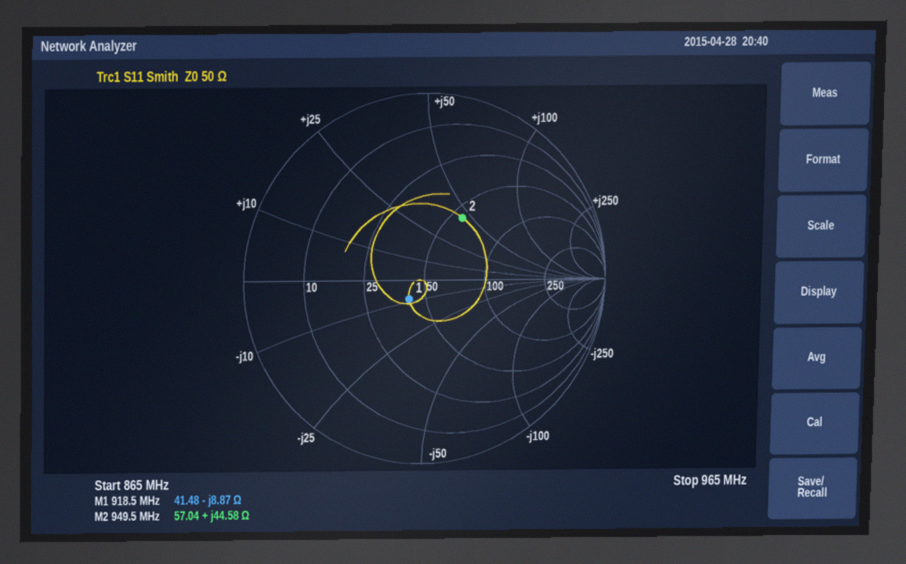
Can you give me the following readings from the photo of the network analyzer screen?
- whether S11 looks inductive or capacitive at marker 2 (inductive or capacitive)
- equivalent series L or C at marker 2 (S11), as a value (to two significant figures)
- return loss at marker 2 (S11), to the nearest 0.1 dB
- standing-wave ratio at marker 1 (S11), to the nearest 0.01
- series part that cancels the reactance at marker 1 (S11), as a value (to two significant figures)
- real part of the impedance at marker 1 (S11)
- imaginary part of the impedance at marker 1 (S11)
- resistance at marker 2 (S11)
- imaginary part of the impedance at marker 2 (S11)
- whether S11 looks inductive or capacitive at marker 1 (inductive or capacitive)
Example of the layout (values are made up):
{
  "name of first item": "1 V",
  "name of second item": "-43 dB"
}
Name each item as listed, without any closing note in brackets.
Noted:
{
  "whether S11 looks inductive or capacitive at marker 2": "inductive",
  "equivalent series L or C at marker 2 (S11), as a value": "7.5 nH",
  "return loss at marker 2 (S11), to the nearest 0.1 dB": "8.2 dB",
  "standing-wave ratio at marker 1 (S11), to the nearest 0.01": "1.31",
  "series part that cancels the reactance at marker 1 (S11), as a value": "1.5 nH",
  "real part of the impedance at marker 1": "41.48 Ω",
  "imaginary part of the impedance at marker 1": "-8.87 Ω",
  "resistance at marker 2": "57.04 Ω",
  "imaginary part of the impedance at marker 2": "+44.58 Ω",
  "whether S11 looks inductive or capacitive at marker 1": "capacitive"
}
